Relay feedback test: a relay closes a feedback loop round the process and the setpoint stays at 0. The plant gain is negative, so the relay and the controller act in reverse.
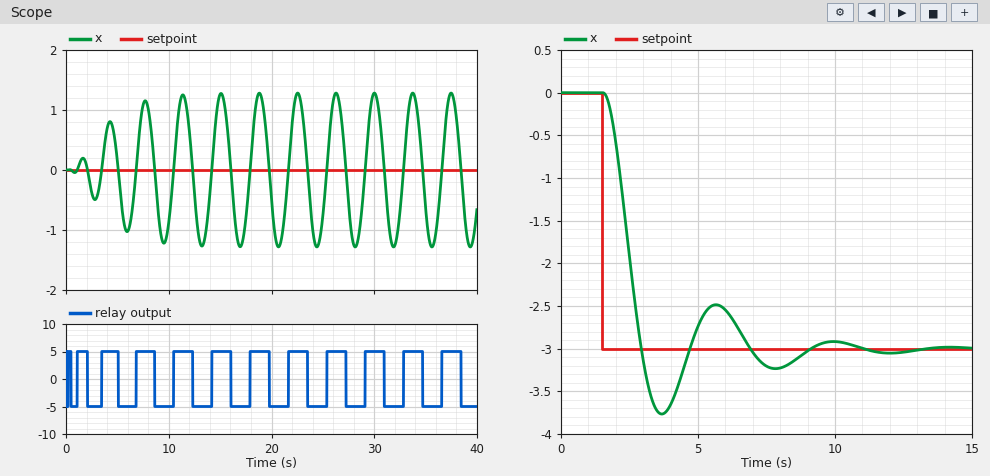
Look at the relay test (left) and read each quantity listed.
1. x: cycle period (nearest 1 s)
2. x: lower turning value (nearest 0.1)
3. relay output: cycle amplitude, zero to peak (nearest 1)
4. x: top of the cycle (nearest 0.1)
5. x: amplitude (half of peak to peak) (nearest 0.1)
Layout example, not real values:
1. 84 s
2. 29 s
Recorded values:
1. 4 s
2. -1.3
3. 5
4. 1.3
5. 1.3
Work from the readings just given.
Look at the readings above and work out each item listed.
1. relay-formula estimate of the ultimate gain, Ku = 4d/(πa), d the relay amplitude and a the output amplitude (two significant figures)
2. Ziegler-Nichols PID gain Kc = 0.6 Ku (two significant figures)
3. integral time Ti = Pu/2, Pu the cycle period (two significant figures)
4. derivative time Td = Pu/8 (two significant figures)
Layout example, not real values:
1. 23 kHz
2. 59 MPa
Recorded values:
1. 4.9
2. 2.9
3. 2.0 s
4. 0.50 s
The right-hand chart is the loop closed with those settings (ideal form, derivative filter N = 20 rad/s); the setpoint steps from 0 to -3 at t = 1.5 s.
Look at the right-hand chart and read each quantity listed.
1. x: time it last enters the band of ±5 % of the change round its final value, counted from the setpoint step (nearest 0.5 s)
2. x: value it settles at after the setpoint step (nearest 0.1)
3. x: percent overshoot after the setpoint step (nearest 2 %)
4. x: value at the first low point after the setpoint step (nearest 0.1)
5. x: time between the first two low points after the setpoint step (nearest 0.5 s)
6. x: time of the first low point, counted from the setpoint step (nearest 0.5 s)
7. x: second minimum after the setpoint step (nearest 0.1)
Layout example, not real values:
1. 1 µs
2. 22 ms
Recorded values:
1. 7.0 s
2. -3.0
3. 26 %
4. -3.8
5. 4.0 s
6. 2.0 s
7. -3.2
